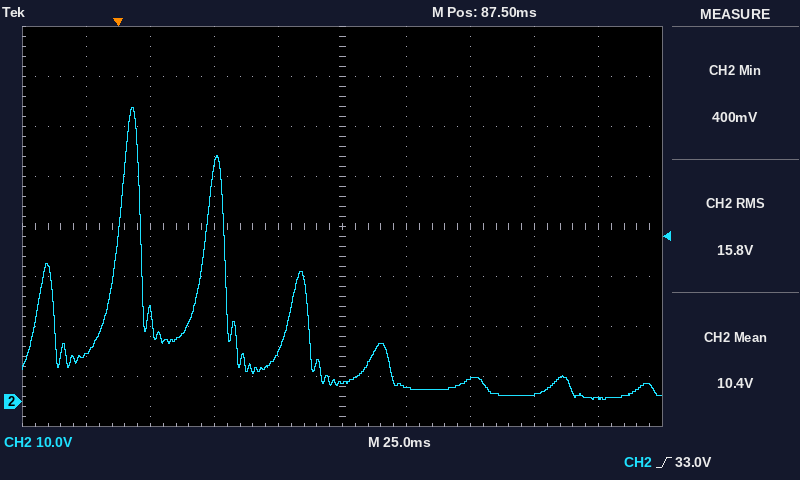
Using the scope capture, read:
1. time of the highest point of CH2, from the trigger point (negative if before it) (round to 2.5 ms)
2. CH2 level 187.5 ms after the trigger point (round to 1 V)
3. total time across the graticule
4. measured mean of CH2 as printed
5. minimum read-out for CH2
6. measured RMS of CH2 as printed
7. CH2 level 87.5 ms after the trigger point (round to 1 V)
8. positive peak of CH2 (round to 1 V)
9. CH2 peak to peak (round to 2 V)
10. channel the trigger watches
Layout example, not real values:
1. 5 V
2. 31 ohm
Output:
1. +5.0 ms
2. 1 V
3. 250 ms
4. 10.4 V
5. 400 mV
6. 15.8 V
7. 4 V
8. 59 V
9. 58 V
10. CH2
